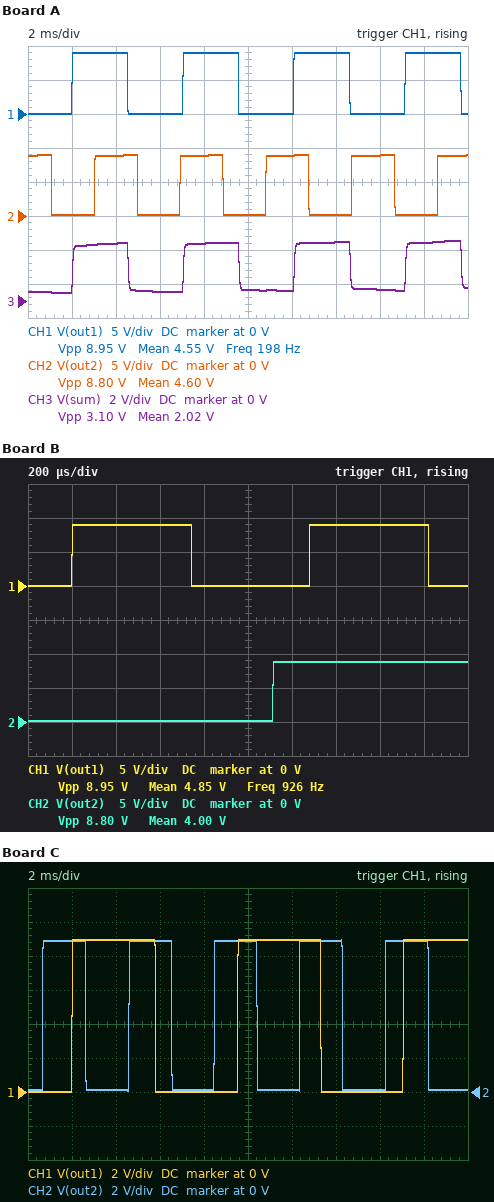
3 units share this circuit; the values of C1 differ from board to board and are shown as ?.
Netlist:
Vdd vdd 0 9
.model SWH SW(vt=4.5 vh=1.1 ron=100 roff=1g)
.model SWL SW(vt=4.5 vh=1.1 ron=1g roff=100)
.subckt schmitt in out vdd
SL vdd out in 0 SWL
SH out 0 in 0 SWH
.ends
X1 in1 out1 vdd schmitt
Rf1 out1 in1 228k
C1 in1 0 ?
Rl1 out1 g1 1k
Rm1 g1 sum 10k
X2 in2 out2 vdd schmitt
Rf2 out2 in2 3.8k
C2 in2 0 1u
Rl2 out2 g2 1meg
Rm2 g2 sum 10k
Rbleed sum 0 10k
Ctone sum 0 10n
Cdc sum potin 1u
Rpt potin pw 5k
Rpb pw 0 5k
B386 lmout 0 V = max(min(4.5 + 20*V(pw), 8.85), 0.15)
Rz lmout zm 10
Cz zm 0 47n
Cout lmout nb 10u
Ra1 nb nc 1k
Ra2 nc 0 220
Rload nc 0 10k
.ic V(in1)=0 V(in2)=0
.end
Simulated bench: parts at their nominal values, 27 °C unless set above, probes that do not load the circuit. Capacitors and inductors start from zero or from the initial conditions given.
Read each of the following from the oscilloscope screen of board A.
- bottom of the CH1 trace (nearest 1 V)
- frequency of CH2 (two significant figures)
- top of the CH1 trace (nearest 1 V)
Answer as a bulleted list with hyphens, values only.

- 0 V
- 260 Hz
- 9 V
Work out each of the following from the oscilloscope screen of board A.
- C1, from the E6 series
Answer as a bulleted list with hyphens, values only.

- 22 nF
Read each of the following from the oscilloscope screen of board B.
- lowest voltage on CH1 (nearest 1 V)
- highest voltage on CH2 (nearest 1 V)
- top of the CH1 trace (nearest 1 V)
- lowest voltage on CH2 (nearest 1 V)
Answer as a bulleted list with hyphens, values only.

- 0 V
- 9 V
- 9 V
- 0 V
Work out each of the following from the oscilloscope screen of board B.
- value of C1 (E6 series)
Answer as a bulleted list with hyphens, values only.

- 4.7 nF
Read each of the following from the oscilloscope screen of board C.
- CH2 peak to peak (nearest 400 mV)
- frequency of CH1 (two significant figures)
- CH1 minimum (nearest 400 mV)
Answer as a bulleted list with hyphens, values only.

- 8.8 V
- 130 Hz
- 0 V
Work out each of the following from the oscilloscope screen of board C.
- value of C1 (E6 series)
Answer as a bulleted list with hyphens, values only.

- 33 nF
